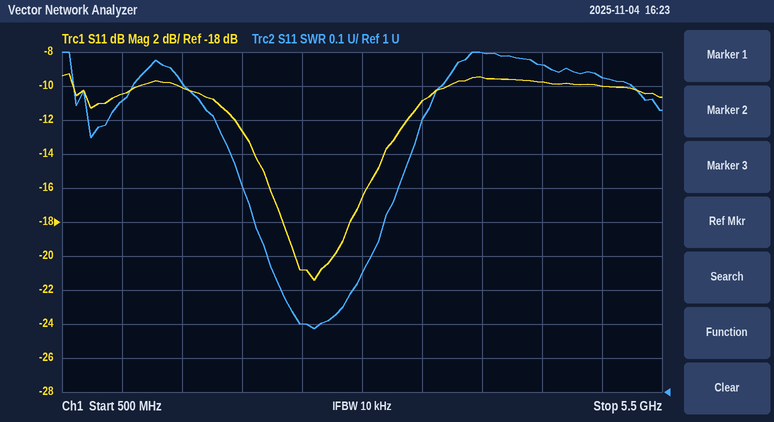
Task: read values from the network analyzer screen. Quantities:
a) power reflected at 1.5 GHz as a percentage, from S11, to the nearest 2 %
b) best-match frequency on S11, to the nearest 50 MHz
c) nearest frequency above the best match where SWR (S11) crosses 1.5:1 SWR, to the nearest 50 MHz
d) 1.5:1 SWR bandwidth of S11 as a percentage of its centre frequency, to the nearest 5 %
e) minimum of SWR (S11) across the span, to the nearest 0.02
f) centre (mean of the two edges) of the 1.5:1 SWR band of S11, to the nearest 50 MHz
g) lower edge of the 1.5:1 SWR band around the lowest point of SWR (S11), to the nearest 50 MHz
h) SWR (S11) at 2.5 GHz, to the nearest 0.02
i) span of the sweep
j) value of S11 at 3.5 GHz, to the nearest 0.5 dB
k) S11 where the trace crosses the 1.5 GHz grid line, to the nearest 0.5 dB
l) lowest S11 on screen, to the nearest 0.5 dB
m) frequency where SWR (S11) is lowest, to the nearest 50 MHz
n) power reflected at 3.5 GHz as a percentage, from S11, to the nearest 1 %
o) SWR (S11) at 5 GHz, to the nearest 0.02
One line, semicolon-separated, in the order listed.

10 %; 2.60 GHz; 3.20 GHz; 40 %; 1.18; 2.65 GHz; 2.10 GHz; 1.20; 5 GHz; -11.0 dB; -10.0 dB; -21.5 dB; 2.60 GHz; 8 %; 1.92
